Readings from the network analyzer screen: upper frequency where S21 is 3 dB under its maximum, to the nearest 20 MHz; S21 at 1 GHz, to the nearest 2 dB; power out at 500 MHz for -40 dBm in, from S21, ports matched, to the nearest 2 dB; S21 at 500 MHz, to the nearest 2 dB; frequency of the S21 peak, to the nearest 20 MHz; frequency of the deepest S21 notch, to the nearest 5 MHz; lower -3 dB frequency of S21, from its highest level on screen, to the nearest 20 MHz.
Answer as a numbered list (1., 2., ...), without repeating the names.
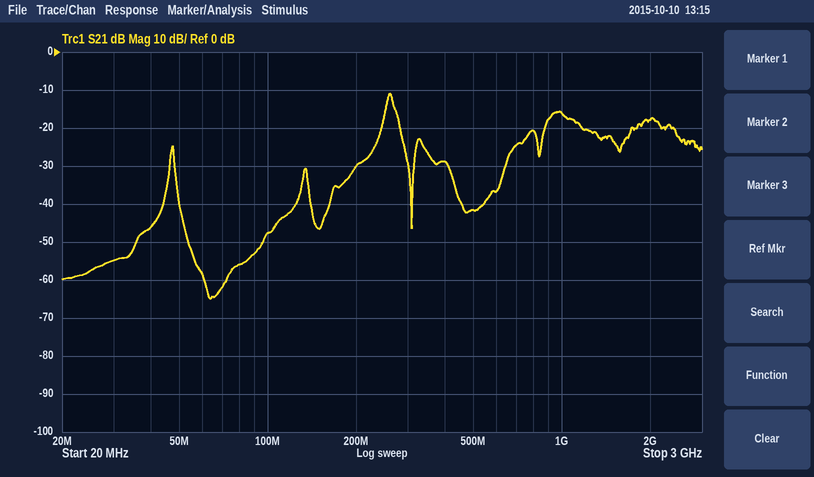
1. 260 MHz
2. -16 dB
3. -82 dBm
4. -42 dB
5. 260 MHz
6. 65 MHz
7. 260 MHz
